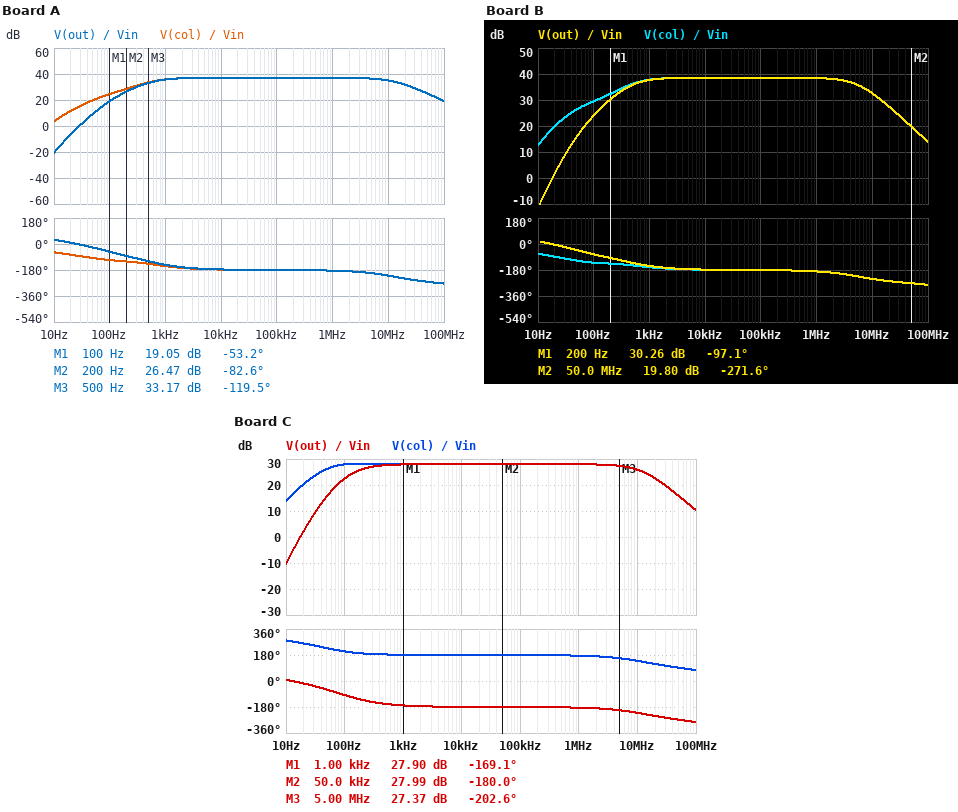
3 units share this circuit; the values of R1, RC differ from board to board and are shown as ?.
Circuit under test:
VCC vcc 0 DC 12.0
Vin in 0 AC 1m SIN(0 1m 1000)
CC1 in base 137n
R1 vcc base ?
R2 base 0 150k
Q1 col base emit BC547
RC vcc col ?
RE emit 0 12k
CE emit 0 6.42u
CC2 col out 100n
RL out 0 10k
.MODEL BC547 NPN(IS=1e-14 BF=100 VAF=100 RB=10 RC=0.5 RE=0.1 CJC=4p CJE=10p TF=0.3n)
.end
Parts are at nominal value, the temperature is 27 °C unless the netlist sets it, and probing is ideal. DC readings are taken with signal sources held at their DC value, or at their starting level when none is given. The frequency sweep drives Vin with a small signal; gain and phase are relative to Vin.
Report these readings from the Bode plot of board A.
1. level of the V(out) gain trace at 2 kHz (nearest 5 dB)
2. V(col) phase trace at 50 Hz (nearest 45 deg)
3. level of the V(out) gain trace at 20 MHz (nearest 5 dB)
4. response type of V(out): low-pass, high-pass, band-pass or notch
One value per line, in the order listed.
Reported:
35 dB
-90 deg
30 dB
band-pass
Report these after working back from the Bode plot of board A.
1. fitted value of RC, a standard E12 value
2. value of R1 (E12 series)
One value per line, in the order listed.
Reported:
8.2 kΩ
150 kΩ
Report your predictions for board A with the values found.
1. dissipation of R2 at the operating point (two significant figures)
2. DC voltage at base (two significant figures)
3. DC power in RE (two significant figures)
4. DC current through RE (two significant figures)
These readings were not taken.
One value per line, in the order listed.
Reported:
220 µW
5.7 V
2.1 mW
420 µA
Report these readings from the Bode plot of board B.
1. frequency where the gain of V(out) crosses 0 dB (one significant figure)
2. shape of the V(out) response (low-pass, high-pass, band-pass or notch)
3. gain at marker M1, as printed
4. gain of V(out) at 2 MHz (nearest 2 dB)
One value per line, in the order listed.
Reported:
20 Hz
band-pass
30.26 dB
38 dB
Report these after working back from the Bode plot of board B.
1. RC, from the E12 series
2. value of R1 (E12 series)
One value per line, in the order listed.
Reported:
22 kΩ
220 kΩ
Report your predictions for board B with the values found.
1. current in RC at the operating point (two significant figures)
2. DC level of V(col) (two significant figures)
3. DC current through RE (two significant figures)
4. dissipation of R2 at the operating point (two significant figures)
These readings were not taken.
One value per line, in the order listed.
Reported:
330 µA
4.8 V
330 µA
140 µW
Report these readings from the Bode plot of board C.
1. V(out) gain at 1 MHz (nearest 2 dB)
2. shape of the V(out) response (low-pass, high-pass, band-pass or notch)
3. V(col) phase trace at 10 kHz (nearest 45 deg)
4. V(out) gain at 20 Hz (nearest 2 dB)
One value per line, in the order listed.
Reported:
28 dB
band-pass
180 deg
2 dB
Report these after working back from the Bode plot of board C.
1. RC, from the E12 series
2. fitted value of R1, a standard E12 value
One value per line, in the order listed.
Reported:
22 kΩ
820 kΩ
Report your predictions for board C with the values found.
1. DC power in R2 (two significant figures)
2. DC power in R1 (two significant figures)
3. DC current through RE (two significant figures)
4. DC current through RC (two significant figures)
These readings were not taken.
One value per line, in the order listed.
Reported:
20 µW
130 µW
96 µA
95 µA
